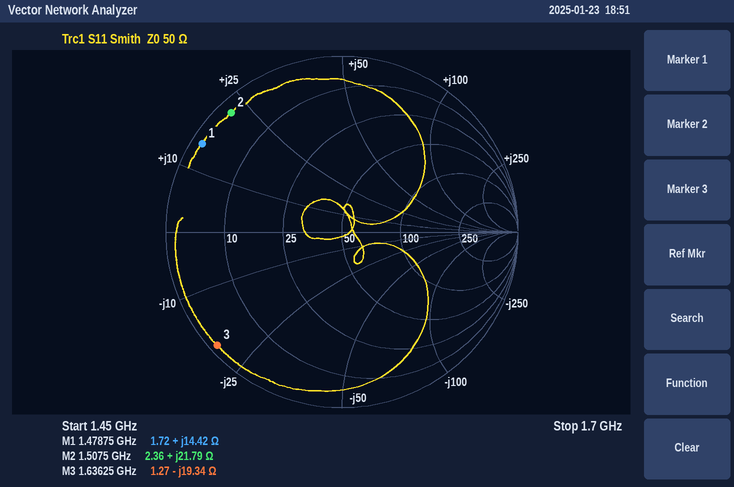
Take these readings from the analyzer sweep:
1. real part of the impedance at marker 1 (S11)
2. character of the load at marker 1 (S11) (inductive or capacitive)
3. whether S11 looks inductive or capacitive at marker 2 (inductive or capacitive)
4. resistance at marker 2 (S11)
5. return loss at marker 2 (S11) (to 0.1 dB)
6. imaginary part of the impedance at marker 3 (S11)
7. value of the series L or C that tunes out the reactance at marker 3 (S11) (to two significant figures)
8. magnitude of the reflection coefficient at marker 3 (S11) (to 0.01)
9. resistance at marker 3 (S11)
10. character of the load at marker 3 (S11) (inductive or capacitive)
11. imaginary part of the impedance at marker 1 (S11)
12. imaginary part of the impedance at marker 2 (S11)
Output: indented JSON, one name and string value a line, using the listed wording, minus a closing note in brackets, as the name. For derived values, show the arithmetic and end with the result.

{
  "real part of the impedance at marker 1": "1.72 Ω",
  "character of the load at marker 1 (S11)": "inductive",
  "whether S11 looks inductive or capacitive at marker 2": "inductive",
  "resistance at marker 2": "2.36 Ω",
  "return loss at marker 2 (S11)": "0.7 dB",
  "imaginary part of the impedance at marker 3": "-19.34 Ω",
  "value of the series L or C that tunes out the reactance at marker 3 (S11)": "L = 19.34 Ω/(2π × 1.63625 GHz) ≈ 1.9 nH",
  "magnitude of the reflection coefficient at marker 3 (S11)": "0.96",
  "resistance at marker 3": "1.27 Ω",
  "character of the load at marker 3 (S11)": "capacitive",
  "imaginary part of the impedance at marker 1": "+14.42 Ω",
  "imaginary part of the impedance at marker 2": "+21.79 Ω"
}
